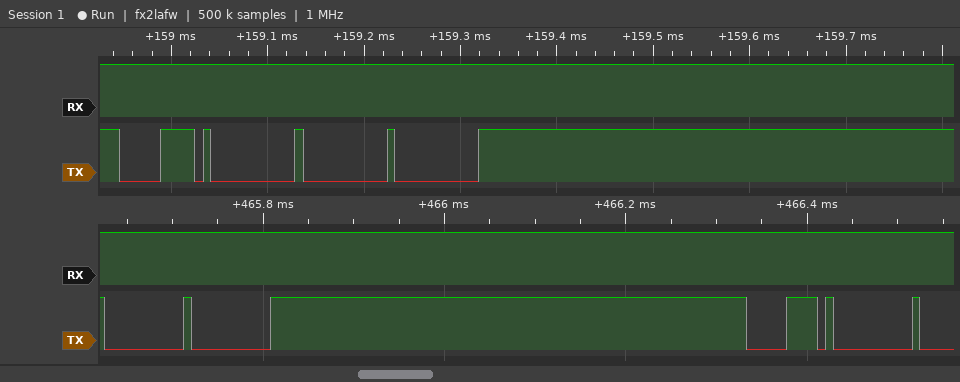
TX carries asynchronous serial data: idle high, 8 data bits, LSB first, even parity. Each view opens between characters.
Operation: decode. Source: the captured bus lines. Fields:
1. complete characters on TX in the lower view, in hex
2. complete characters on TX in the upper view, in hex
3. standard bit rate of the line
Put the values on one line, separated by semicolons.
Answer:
00, 00, F0, 00; F0, 00, 00, 00; 115200 baud
